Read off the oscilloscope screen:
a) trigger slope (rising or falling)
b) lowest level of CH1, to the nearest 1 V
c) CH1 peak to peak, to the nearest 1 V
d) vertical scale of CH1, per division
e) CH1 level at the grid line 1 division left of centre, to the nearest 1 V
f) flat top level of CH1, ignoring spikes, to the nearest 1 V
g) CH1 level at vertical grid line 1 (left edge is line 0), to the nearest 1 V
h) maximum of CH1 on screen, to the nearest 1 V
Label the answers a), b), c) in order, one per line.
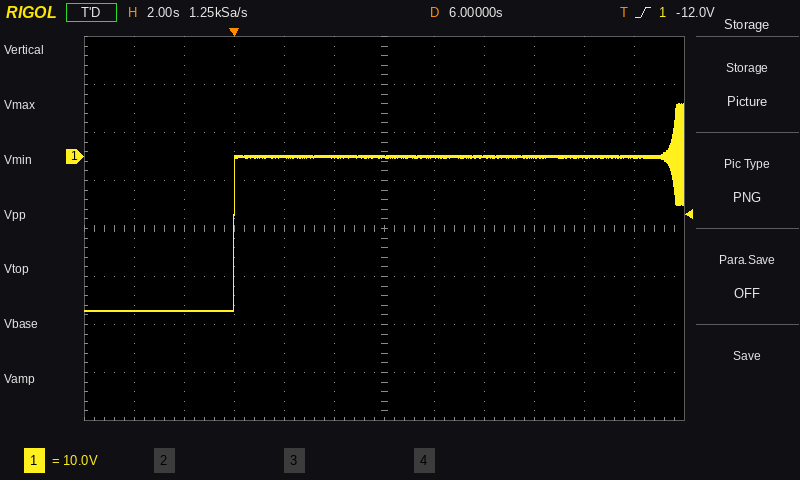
a) rising
b) -32 V
c) 43 V
d) 10 V
e) 0 V
f) 0 V
g) -32 V
h) 11 V
